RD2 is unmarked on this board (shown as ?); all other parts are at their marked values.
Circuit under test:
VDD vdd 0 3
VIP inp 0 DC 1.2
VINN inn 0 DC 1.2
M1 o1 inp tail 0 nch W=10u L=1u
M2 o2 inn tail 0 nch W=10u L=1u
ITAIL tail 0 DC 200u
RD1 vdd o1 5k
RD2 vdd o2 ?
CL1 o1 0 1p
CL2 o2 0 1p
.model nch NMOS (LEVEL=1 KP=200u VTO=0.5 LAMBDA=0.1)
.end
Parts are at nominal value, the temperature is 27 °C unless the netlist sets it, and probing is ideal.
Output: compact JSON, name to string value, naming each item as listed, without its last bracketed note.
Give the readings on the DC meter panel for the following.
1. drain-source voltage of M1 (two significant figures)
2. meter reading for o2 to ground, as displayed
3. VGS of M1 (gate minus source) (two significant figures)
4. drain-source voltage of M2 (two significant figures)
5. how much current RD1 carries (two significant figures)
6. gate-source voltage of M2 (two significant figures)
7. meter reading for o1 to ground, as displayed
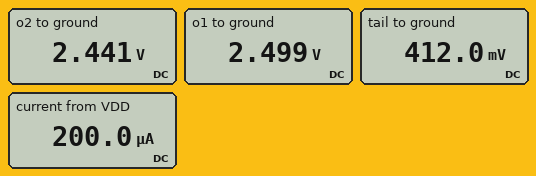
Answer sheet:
{"drain-source voltage of M1": "2.1 V", "meter reading for o2 to ground, as displayed": "2.441 V", "VGS of M1 (gate minus source)": "790 mV", "drain-source voltage of M2": "2.0 V", "how much current RD1 carries": "100 µA", "gate-source voltage of M2": "790 mV", "meter reading for o1 to ground, as displayed": "2.499 V"}
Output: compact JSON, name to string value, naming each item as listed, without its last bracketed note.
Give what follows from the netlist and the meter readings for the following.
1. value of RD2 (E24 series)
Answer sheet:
{"value of RD2": "5.6 kΩ"}
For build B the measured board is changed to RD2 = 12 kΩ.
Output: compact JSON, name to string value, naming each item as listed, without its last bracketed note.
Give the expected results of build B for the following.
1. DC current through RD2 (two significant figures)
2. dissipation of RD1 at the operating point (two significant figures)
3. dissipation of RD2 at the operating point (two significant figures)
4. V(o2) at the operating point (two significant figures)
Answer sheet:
{"DC current through RD2": "97 µA", "dissipation of RD1 at the operating point": "53 µW", "dissipation of RD2 at the operating point": "110 µW", "V(o2) at the operating point": "1.8 V"}
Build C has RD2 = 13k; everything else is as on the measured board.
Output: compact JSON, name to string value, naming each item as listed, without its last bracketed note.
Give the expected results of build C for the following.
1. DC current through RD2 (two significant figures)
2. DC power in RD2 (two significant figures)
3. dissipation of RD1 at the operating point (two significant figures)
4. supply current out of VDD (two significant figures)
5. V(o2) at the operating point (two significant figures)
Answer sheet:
{"DC current through RD2": "97 µA", "DC power in RD2": "120 µW", "dissipation of RD1 at the operating point": "53 µW", "supply current out of VDD": "200 µA", "V(o2) at the operating point": "1.7 V"}
